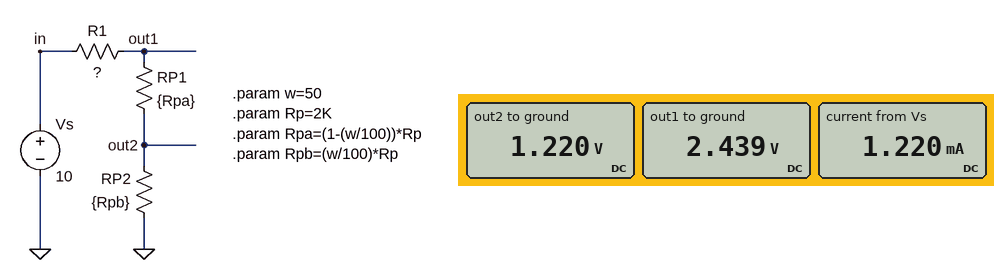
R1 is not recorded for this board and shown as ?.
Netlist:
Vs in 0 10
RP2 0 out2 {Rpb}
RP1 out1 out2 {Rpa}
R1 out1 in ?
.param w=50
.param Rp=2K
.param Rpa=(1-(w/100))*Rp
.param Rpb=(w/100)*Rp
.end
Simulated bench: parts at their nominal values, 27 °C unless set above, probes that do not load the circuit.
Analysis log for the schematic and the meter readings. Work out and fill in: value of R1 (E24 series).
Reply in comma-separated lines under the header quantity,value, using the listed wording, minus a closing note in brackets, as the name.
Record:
quantity,value
value of R1,6.2 kΩ
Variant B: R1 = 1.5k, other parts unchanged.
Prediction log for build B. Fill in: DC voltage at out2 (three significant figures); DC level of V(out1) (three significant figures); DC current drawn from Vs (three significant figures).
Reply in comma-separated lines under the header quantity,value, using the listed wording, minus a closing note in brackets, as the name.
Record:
quantity,value
DC voltage at out2,2.86 V
DC level of V(out1),5.71 V
DC current drawn from Vs,2.86 mA
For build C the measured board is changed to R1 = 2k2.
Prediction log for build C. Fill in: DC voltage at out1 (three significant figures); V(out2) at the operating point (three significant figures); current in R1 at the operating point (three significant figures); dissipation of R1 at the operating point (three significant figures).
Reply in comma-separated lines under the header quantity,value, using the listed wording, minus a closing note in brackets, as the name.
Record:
quantity,value
DC voltage at out1,4.76 V
V(out2) at the operating point,2.38 V
current in R1 at the operating point,2.38 mA
dissipation of R1 at the operating point,12.5 mW
